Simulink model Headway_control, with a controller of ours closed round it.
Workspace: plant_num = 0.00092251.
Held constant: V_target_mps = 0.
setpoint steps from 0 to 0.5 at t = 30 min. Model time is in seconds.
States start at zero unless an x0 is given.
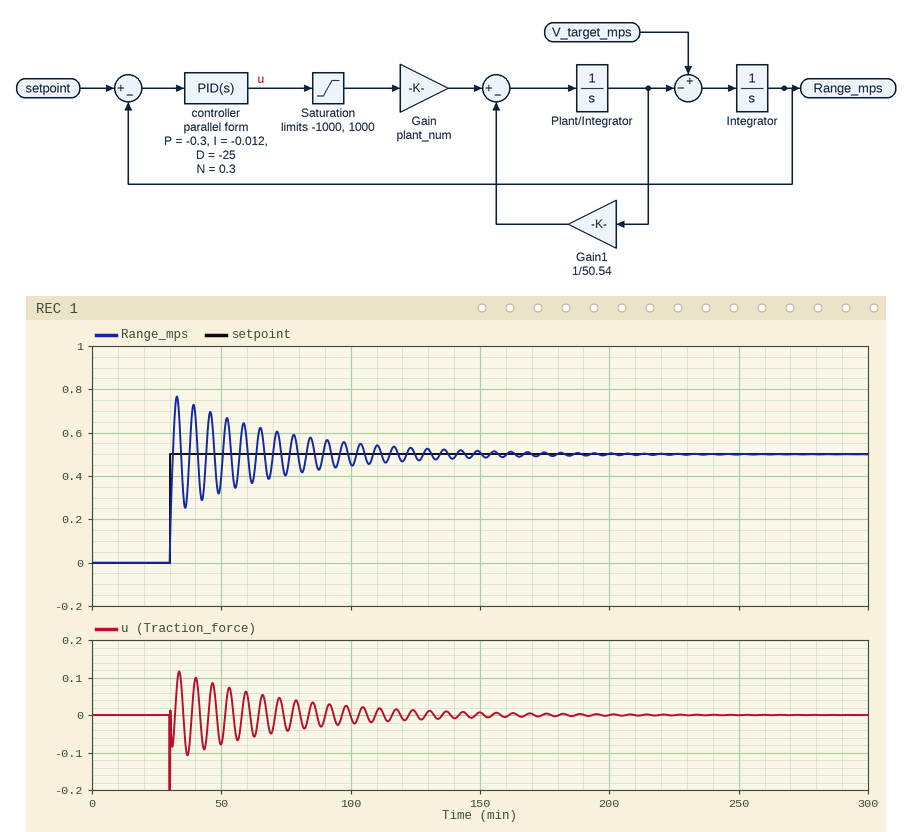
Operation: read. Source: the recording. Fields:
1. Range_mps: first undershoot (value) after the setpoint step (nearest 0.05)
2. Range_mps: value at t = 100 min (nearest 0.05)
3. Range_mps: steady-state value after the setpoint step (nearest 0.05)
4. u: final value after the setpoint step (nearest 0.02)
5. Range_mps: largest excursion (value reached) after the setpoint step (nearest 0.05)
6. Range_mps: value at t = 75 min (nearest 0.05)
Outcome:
0.25
0.45
0.50
0.00
0.75
0.40
